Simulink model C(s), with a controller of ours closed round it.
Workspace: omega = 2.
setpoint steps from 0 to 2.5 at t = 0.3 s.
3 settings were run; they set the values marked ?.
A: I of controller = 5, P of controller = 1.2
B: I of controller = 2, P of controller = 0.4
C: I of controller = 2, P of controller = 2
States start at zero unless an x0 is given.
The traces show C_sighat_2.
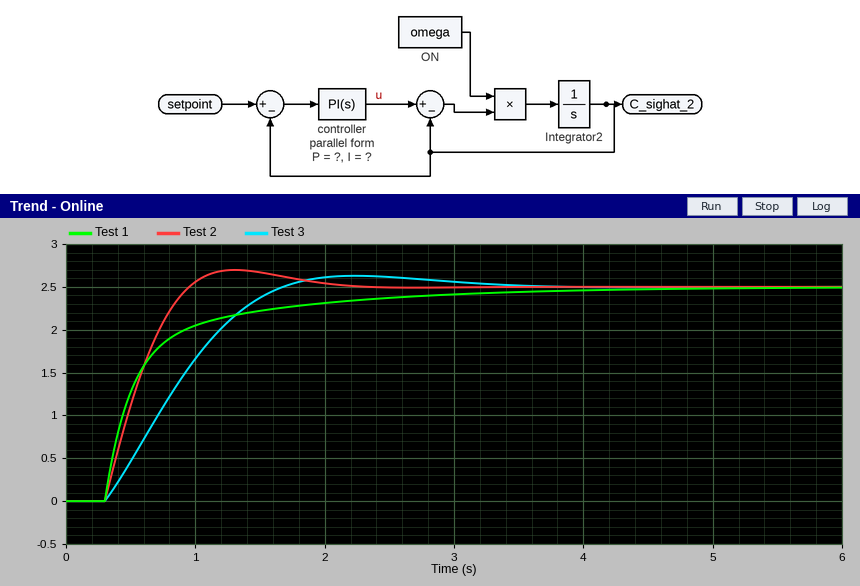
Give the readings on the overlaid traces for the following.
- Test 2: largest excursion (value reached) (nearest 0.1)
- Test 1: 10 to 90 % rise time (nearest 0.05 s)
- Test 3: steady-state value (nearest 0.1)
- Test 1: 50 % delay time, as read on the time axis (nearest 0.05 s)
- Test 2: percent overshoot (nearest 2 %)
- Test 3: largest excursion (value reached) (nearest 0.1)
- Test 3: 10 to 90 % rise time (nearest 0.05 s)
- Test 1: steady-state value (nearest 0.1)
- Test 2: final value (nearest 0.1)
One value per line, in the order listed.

2.7
1.30 s
2.5
0.50 s
8 %
2.6
0.95 s
2.5
2.5
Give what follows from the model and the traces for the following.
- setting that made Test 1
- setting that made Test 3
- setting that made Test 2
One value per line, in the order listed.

C
B
A
